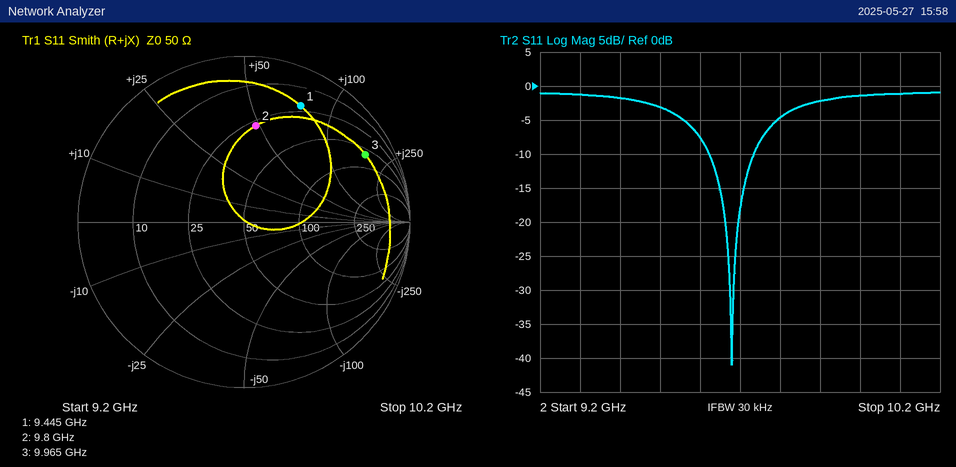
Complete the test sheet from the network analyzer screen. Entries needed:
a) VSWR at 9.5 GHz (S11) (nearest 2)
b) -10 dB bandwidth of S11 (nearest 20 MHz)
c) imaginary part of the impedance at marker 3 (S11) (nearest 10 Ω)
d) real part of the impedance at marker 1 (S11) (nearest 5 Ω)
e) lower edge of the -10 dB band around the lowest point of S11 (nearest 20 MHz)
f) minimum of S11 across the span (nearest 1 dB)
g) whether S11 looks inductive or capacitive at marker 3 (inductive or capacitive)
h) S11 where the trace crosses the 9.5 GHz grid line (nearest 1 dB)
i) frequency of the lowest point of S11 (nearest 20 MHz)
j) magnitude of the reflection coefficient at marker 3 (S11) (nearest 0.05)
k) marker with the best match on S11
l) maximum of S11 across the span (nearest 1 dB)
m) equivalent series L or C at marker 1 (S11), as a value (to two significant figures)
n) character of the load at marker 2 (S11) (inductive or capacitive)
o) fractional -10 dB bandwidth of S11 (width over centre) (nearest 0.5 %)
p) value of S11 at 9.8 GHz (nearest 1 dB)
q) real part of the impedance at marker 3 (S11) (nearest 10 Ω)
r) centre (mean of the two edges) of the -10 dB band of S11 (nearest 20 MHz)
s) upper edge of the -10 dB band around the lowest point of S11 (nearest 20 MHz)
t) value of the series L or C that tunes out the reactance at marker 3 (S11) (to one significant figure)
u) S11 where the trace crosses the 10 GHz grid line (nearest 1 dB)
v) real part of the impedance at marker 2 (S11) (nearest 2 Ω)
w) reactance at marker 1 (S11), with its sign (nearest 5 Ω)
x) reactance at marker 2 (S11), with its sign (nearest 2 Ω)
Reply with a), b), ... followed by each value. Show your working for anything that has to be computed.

a) |Γ| = 10^(-3/20) = 0.7079; VSWR = (1 + 0.7079)/(1 − 0.7079) ≈ 6
b) 9.74 GHz − 9.62 GHz = 120 MHz
c) +170 Ω
d) 20 Ω
e) 9.62 GHz
f) -41 dB
g) inductive
h) -3 dB
i) 9.68 GHz
j) 0.85
k) marker 2
l) -1 dB
m) L = 75 Ω/(2π × 9.445 GHz) ≈ 1.3 nH
n) inductive
o) 120 MHz / 9.68 GHz ≈ 1.24 %, so 1.0 % to the nearest 0.5 %
p) -5 dB
q) 60 Ω
r) 9.68 GHz
s) 9.74 GHz
t) C = 1/(2π × 9.965 GHz × 170 Ω) ≈ 93.9 fF, so 90 fF to one significant figure
u) -1 dB
v) 28 Ω
w) +75 Ω
x) +48 Ω
